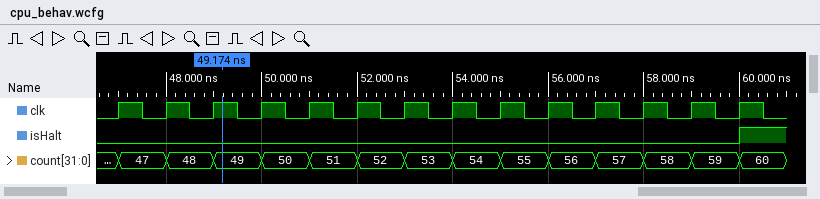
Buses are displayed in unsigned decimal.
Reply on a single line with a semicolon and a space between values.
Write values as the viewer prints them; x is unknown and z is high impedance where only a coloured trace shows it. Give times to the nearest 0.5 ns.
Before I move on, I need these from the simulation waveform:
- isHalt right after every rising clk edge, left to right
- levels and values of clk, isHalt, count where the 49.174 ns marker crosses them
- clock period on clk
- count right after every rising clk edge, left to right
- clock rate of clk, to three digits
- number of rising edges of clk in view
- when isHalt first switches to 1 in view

0 0 0 0 0 0 0 0 0 0 0 0 0 1; clk=1, isHalt=0, count=49; 1 ns; 47, 48, 49, 50, 51, 52, 53, 54, 55, 56, 57, 58, 59, 60; 1.00 GHz; 14; 60 ns
